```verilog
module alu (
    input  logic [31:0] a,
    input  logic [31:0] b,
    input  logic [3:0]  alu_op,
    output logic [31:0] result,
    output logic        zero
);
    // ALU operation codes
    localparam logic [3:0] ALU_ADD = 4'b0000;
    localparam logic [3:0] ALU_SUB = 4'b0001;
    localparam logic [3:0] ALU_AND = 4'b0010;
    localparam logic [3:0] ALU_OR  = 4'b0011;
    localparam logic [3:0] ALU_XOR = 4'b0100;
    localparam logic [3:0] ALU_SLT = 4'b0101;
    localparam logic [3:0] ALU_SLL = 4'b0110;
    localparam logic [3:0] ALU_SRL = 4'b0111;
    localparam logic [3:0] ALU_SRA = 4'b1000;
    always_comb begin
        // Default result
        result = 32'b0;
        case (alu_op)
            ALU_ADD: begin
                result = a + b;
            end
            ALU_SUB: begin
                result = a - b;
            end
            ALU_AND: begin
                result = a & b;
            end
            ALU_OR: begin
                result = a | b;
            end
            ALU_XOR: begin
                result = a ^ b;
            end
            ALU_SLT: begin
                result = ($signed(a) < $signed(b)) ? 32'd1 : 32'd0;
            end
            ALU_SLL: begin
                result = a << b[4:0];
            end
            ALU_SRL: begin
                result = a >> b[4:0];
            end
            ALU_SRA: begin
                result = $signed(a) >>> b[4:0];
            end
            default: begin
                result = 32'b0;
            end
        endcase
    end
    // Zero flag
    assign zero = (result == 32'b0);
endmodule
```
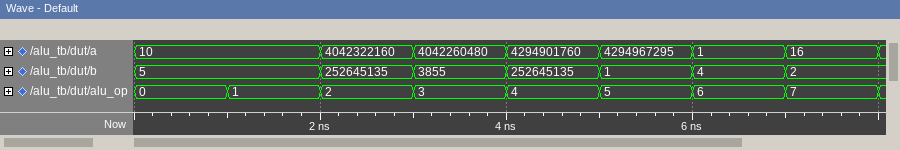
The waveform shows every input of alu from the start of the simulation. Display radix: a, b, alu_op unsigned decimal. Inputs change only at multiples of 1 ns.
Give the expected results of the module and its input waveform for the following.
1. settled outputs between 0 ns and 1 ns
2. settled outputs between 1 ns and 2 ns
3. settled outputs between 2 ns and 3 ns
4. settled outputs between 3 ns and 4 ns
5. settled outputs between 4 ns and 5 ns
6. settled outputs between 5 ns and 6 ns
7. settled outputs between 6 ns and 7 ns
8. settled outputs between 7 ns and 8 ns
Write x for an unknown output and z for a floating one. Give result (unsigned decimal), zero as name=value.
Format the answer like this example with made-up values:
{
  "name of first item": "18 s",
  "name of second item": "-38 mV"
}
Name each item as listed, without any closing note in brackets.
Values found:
{
  "settled outputs between 0 ns and 1 ns": "result=15, zero=0",
  "settled outputs between 1 ns and 2 ns": "result=5, zero=0",
  "settled outputs between 2 ns and 3 ns": "result=0, zero=1",
  "settled outputs between 3 ns and 4 ns": "result=4042264335, zero=0",
  "settled outputs between 4 ns and 5 ns": "result=4042264335, zero=0",
  "settled outputs between 5 ns and 6 ns": "result=1, zero=0",
  "settled outputs between 6 ns and 7 ns": "result=16, zero=0",
  "settled outputs between 7 ns and 8 ns": "result=4, zero=0"
}
